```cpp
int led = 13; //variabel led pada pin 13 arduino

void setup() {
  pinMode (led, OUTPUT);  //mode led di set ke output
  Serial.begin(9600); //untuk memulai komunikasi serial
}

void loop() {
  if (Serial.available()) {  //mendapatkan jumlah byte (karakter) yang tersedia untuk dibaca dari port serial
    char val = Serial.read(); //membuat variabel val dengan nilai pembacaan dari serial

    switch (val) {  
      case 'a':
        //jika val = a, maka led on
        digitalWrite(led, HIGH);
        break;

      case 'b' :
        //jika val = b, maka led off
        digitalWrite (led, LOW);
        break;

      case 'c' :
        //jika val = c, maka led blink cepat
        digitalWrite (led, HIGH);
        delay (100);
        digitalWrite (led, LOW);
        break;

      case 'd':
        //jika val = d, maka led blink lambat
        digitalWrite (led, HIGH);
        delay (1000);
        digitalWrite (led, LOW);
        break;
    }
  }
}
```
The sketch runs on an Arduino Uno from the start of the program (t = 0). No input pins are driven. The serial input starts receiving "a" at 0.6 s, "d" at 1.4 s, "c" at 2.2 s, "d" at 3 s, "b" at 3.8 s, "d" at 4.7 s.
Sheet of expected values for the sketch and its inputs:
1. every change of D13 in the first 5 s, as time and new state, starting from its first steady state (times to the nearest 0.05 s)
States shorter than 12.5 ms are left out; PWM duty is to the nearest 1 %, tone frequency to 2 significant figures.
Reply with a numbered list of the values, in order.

1. 0 s low; 0.6 s high; 2.5 s low; 3 s high; 4 s low; 4.7 s high
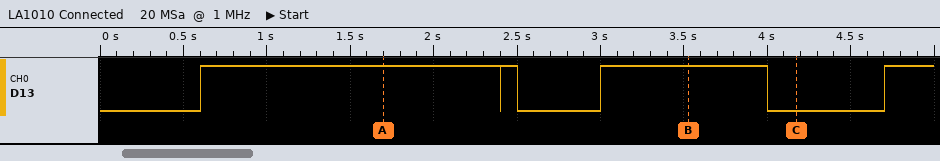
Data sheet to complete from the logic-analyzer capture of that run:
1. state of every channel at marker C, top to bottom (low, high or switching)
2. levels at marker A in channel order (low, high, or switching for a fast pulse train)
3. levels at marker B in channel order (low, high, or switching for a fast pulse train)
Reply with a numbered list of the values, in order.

1. D13 low
2. D13 high
3. D13 high
